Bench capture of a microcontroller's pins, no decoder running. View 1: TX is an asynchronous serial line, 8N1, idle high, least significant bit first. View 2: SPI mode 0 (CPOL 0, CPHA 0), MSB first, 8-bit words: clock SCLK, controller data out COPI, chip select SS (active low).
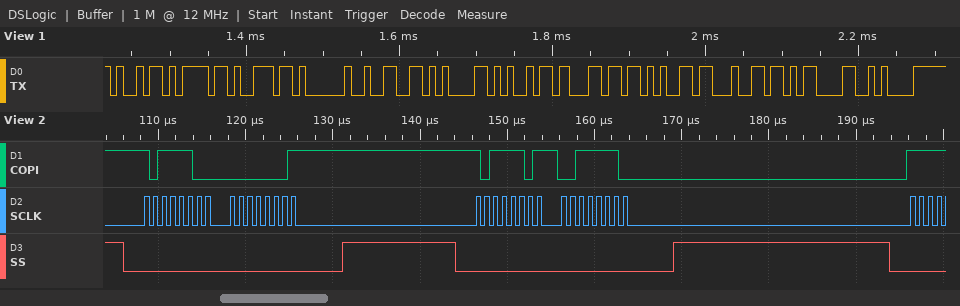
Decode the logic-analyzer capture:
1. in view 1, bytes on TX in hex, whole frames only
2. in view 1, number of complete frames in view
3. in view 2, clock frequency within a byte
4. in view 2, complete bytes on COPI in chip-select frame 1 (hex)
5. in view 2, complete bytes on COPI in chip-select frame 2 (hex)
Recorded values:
69 6F 6E 20 66 61 69 6C 65 64 0D 0A
12
1 MHz
BC 01
BD 3E
